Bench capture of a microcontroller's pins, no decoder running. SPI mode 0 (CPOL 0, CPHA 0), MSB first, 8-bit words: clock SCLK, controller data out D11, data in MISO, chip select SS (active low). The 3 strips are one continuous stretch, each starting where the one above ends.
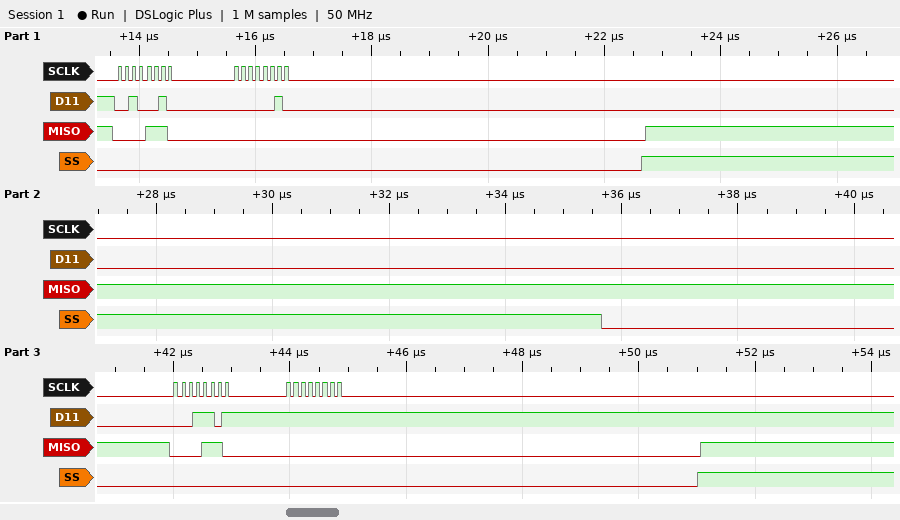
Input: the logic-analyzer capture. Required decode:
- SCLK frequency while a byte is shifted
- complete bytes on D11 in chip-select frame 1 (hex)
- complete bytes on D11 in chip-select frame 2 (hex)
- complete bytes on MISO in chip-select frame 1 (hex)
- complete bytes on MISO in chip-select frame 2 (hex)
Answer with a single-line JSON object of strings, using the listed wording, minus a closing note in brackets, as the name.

{"SCLK frequency while a byte is shifted": "8 MHz", "complete bytes on D11 in chip-select frame 1": "22 02", "complete bytes on D11 in chip-select frame 2": "1D FF", "complete bytes on MISO in chip-select frame 1": "0E 00", "complete bytes on MISO in chip-select frame 2": "0E 00"}
